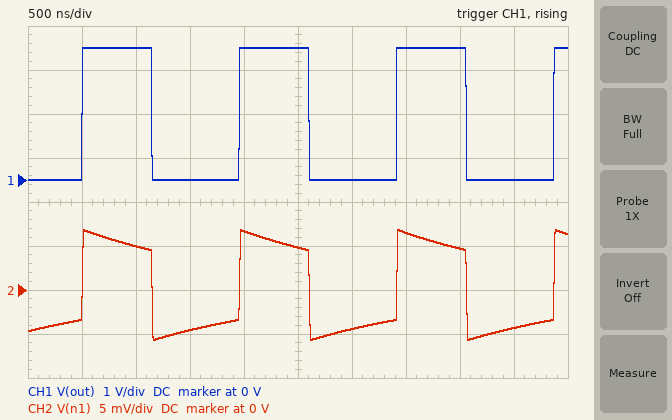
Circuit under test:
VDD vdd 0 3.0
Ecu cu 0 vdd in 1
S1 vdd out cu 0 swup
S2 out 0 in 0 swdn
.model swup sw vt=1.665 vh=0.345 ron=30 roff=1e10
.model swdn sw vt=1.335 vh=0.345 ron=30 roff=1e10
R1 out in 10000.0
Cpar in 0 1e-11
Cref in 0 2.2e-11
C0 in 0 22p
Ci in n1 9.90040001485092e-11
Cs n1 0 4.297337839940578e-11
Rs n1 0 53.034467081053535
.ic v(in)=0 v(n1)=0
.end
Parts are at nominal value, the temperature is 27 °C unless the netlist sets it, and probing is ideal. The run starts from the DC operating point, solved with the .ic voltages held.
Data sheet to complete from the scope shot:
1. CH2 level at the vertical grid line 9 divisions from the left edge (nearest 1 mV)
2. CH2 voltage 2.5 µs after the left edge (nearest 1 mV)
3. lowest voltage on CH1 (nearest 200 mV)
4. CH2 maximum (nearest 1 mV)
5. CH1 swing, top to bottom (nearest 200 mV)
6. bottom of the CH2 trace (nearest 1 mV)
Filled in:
-4 mV
5 mV
0 V
7 mV
3.0 V
-6 mV
